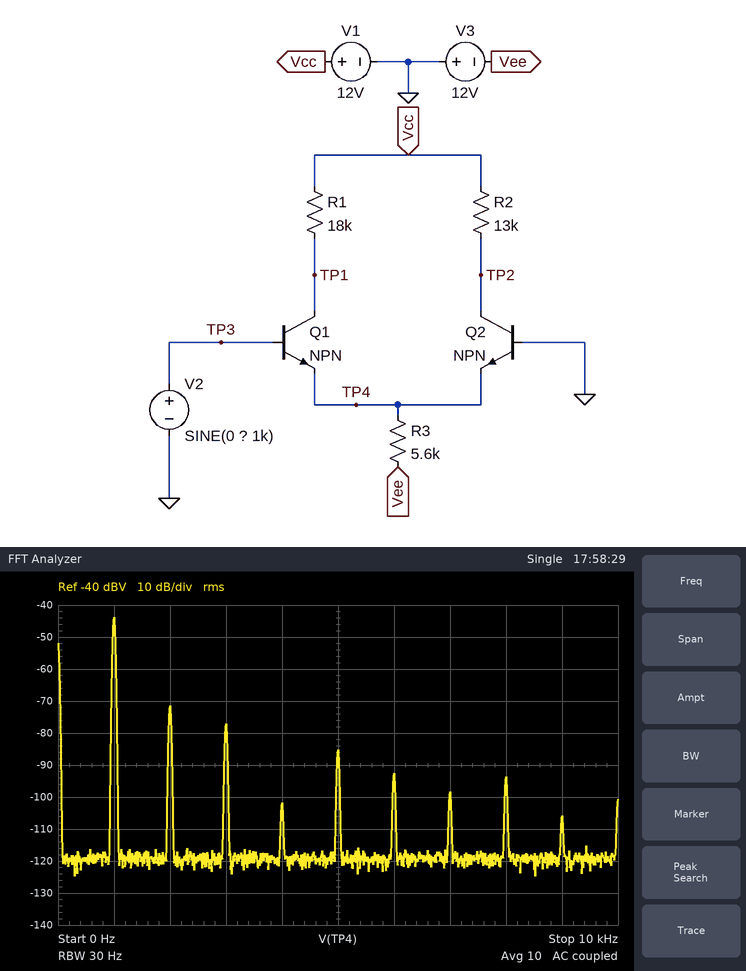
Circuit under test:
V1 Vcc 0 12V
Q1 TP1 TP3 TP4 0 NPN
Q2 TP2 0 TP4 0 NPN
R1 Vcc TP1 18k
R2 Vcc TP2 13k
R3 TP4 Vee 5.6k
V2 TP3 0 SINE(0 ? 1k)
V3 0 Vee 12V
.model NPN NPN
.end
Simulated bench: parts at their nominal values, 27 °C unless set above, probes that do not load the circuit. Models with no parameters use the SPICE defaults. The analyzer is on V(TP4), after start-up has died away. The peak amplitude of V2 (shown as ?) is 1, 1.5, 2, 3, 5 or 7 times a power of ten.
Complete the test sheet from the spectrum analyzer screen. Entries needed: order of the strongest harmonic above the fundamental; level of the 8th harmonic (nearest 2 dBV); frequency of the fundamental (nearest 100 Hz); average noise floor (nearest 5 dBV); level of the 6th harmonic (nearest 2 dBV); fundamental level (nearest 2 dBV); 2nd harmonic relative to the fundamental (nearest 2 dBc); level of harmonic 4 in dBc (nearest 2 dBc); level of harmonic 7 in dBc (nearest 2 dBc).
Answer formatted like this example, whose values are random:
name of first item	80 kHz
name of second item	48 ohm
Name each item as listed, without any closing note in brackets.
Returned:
order of the strongest harmonic above the fundamental	2
level of the 8th harmonic	-94 dBV
frequency of the fundamental	1.0 kHz
average noise floor	-120 dBV
level of the 6th harmonic	-92 dBV
fundamental level	-44 dBV
2nd harmonic relative to the fundamental	-28 dBc
level of harmonic 4 in dBc	-58 dBc
level of harmonic 7 in dBc	-54 dBc
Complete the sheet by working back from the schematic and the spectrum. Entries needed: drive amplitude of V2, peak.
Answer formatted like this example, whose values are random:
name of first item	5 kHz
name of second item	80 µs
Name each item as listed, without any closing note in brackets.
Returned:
drive amplitude of V2, peak	20 mV
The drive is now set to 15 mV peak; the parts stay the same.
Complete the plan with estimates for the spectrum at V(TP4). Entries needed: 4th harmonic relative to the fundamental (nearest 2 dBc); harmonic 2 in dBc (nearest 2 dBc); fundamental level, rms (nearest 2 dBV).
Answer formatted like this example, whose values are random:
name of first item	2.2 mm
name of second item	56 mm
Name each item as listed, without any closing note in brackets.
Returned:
4th harmonic relative to the fundamental	-46 dBc
harmonic 2 in dBc	-32 dBc
fundamental level, rms	-46 dBV
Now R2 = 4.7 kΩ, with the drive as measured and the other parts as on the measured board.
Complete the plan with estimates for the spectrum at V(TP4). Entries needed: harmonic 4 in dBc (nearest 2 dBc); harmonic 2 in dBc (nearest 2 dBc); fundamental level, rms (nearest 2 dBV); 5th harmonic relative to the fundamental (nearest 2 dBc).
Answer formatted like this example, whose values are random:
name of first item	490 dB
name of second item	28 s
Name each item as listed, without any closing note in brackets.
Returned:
harmonic 4 in dBc	-40 dBc
harmonic 2 in dBc	-20 dBc
fundamental level, rms	-46 dBV
5th harmonic relative to the fundamental	-46 dBc
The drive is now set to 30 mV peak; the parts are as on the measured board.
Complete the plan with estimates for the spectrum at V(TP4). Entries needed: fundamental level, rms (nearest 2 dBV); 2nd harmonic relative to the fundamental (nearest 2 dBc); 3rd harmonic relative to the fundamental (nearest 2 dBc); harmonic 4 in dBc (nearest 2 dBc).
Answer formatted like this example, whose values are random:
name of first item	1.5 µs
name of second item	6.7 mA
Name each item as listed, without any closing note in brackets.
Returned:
fundamental level, rms	-40 dBV
2nd harmonic relative to the fundamental	-26 dBc
3rd harmonic relative to the fundamental	-50 dBc
harmonic 4 in dBc	-54 dBc
